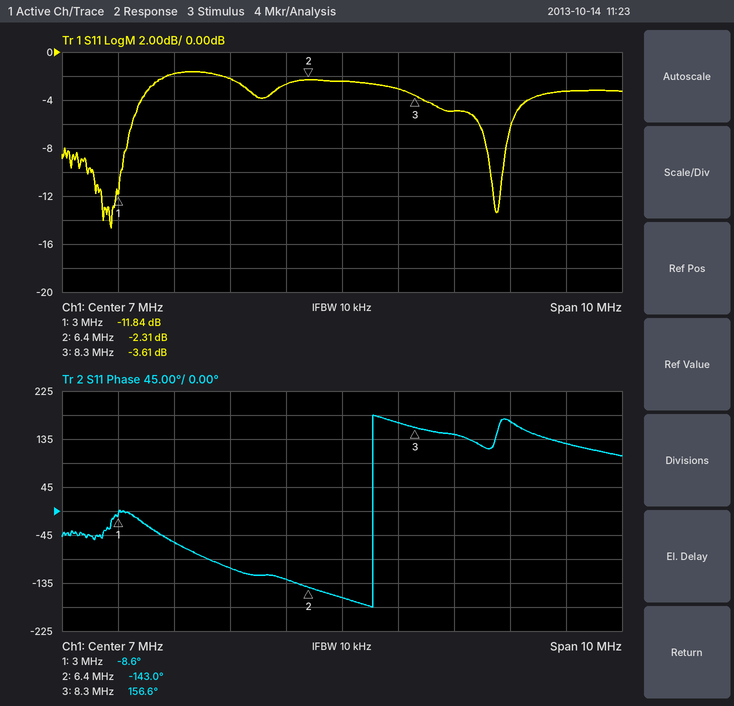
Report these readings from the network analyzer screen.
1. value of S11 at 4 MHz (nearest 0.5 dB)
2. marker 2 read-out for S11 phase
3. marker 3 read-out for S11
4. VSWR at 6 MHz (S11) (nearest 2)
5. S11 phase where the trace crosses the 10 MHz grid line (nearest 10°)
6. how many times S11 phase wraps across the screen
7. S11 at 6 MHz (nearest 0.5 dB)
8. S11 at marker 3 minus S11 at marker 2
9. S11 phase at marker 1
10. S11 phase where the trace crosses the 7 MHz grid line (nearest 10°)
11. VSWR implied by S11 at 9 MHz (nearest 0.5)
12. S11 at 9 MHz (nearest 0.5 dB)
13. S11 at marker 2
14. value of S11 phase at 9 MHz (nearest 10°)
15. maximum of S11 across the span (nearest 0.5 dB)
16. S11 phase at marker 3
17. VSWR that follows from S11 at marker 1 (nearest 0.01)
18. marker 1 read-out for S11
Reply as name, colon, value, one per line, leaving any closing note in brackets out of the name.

value of S11 at 4 MHz: -2.0 dB
marker 2 read-out for S11 phase: -143.0°
marker 3 read-out for S11: -3.61 dB
VSWR at 6 MHz (S11): 6
S11 phase where the trace crosses the 10 MHz grid line: 170°
how many times S11 phase wraps across the screen: 1
S11 at 6 MHz: -2.5 dB
S11 at marker 3 minus S11 at marker 2: -1.30 dB
S11 phase at marker 1: -8.6°
S11 phase where the trace crosses the 7 MHz grid line: -160°
VSWR implied by S11 at 9 MHz: 3.5
S11 at 9 MHz: -5.0 dB
S11 at marker 2: -2.31 dB
value of S11 phase at 9 MHz: 140°
maximum of S11 across the span: -1.5 dB
S11 phase at marker 3: 156.6°
VSWR that follows from S11 at marker 1: 1.69
marker 1 read-out for S11: -11.84 dB
